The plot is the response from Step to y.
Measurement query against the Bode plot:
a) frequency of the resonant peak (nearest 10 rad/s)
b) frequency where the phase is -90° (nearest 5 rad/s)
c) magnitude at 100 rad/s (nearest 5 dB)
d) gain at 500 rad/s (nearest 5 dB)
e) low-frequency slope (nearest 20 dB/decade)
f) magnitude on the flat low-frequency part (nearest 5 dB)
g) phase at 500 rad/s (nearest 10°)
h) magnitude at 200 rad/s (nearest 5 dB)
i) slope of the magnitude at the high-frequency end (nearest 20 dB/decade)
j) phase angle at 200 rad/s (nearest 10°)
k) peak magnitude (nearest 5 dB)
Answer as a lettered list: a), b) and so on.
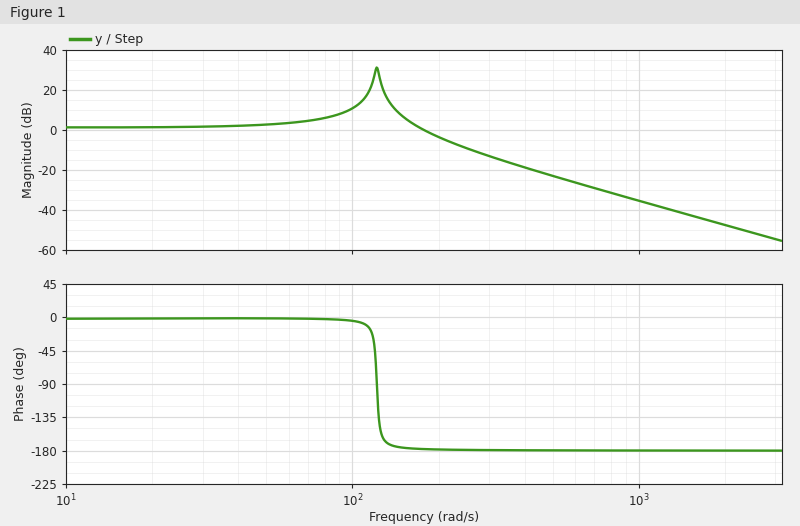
a) 120 rad/s
b) 120 rad/s
c) 10 dB
d) -25 dB
e) 0 dB/decade
f) 0 dB
g) -180°
h) -5 dB
i) -40 dB/decade
j) -180°
k) 30 dB
